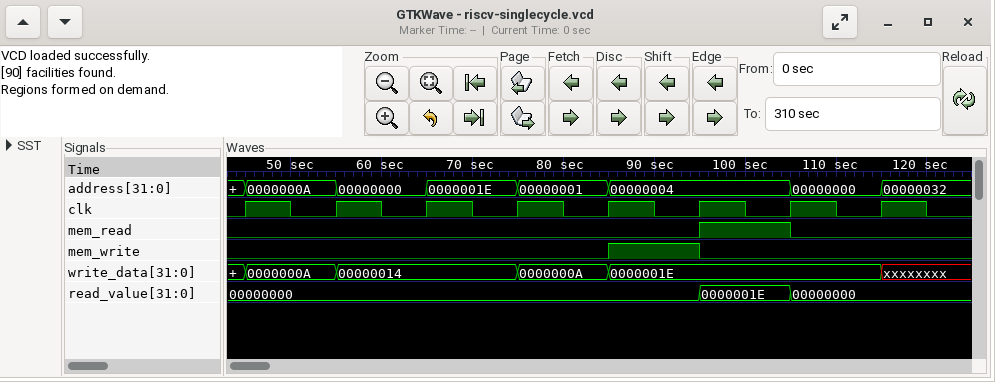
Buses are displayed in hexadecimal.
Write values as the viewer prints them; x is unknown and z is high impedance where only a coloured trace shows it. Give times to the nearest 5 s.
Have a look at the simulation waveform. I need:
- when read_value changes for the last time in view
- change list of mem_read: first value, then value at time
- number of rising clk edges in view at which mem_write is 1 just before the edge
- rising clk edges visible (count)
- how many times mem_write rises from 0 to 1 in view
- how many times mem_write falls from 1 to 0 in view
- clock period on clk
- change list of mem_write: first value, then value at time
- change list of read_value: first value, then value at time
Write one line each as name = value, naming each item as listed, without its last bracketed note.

when read_value changes for the last time in view = 105 s
change list of mem_read: first value, then value at time = 0, 1 at 95 s, 0 at 105 s
number of rising clk edges in view at which mem_write is 1 just before the edge = 1
rising clk edges visible = 8
how many times mem_write rises from 0 to 1 in view = 1
how many times mem_write falls from 1 to 0 in view = 1
clock period on clk = 10 s
change list of mem_write: first value, then value at time = 0, 1 at 85 s, 0 at 95 s
change list of read_value: first value, then value at time = 00000000, 0000001E at 95 s, 00000000 at 105 s
